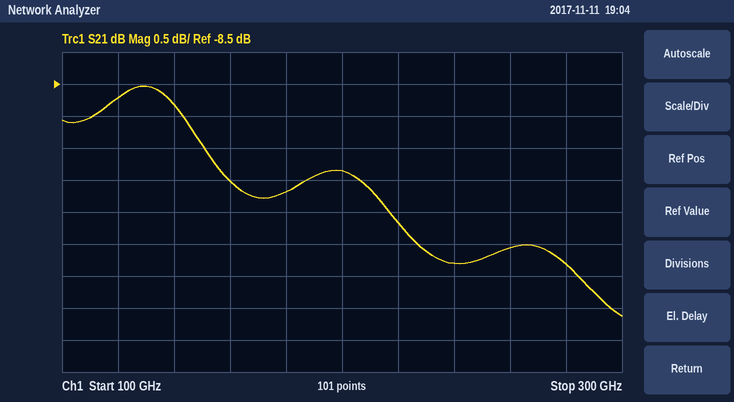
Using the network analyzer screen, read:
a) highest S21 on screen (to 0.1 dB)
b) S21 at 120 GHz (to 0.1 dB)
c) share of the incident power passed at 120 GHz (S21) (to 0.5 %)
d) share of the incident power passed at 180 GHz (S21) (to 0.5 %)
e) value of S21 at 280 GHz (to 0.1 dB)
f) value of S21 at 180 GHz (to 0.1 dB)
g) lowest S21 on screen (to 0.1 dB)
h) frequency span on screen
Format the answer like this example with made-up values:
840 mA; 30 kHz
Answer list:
-8.5 dB; -8.7 dB; 13.5 %; 9.5 %; -11.3 dB; -10.2 dB; -12.1 dB; 200 GHz
